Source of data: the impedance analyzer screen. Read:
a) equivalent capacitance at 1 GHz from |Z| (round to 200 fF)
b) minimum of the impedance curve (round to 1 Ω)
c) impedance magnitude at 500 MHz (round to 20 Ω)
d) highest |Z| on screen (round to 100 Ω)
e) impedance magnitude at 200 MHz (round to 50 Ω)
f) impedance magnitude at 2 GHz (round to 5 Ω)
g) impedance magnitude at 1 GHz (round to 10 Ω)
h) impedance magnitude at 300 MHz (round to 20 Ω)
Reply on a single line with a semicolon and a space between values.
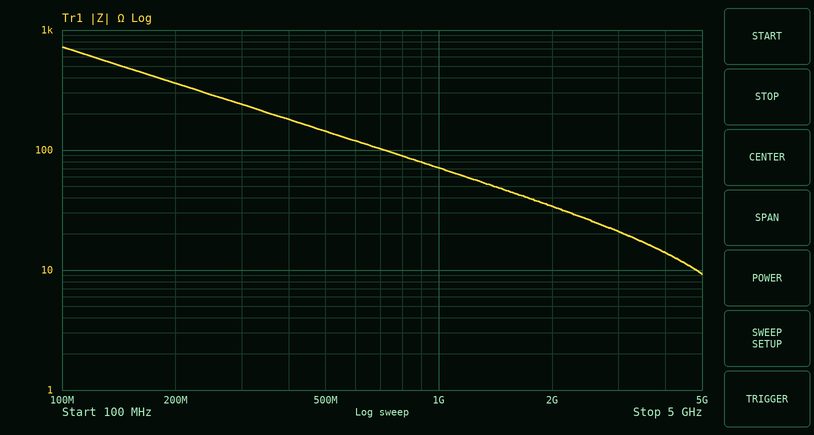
2.2 pF; 9 Ω; 140 Ω; 700 Ω; 350 Ω; 35 Ω; 70 Ω; 240 Ω
